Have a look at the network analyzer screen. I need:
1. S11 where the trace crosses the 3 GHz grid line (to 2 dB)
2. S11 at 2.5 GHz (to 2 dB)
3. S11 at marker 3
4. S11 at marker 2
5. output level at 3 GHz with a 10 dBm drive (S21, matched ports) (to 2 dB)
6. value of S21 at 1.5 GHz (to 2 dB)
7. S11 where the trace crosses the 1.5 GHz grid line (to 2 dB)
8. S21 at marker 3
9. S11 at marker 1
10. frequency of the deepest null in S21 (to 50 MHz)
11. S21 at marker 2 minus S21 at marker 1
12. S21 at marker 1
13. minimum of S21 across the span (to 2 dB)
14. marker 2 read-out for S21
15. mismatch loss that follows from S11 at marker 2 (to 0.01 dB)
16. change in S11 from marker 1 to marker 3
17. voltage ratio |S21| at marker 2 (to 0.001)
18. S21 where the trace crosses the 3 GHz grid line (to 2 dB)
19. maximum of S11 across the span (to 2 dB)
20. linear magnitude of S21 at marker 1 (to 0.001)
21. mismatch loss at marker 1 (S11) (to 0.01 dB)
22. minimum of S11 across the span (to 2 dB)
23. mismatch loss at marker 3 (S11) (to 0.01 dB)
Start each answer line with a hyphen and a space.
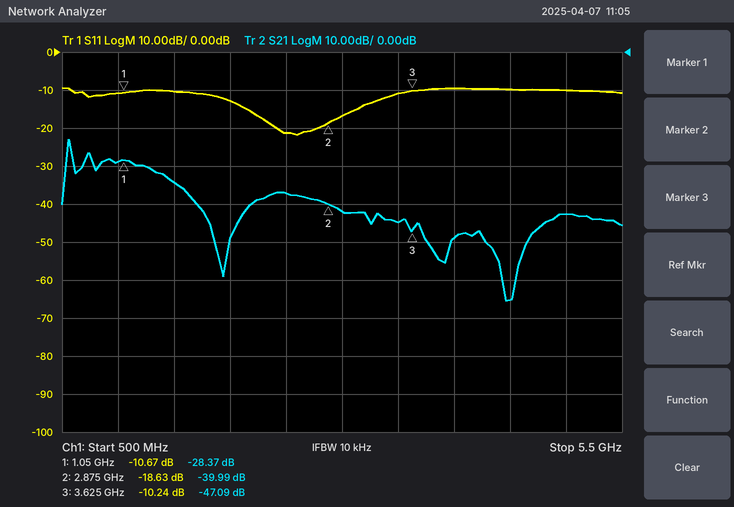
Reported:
- -16 dB
- -22 dB
- -10.24 dB
- -18.63 dB
- -32 dBm
- -34 dB
- -10 dB
- -47.09 dB
- -10.67 dB
- 4.45 GHz
- -11.62 dB
- -28.37 dB
- -66 dB
- -39.99 dB
- 0.06 dB
- 0.43 dB
- 0.010
- -42 dB
- -10 dB
- 0.038
- 0.39 dB
- -22 dB
- 0.43 dB
